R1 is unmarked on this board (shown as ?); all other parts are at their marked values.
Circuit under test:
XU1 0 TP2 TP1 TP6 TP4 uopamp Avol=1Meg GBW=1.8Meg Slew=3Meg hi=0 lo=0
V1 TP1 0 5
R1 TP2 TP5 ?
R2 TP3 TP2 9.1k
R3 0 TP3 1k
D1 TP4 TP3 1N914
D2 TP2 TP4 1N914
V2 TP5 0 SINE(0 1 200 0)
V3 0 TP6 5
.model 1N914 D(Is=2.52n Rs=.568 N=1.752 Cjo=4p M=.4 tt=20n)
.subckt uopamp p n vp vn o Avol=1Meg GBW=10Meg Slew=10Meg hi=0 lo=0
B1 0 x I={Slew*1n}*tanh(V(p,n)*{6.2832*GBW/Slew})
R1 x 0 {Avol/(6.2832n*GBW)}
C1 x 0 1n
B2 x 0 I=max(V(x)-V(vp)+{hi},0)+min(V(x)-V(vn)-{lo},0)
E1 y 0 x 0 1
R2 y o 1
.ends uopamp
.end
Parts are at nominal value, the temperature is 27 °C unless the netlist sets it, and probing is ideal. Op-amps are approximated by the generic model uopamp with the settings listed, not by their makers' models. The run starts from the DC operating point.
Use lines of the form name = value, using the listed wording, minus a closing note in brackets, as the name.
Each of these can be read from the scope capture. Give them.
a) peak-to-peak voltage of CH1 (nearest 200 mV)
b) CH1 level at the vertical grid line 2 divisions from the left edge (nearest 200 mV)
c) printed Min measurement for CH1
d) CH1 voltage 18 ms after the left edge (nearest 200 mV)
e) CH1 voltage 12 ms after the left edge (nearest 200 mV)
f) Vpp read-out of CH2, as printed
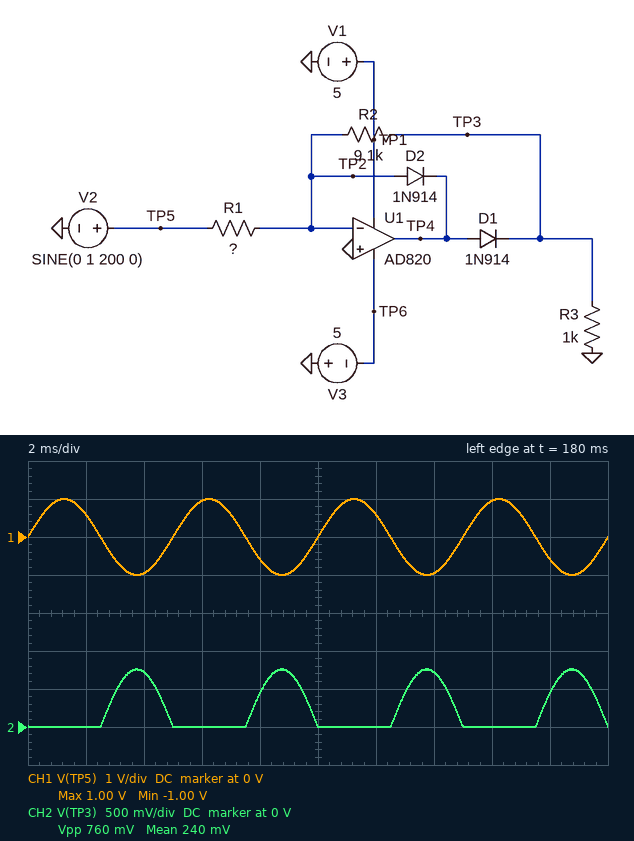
peak-to-peak voltage of CH1 = 2.0 V
CH1 level at the vertical grid line 2 divisions from the left edge = -1.0 V
printed Min measurement for CH1 = -1.00 V
CH1 voltage 18 ms after the left edge = -600 mV
CH1 voltage 12 ms after the left edge = 600 mV
Vpp read-out of CH2, as printed = 760 mV
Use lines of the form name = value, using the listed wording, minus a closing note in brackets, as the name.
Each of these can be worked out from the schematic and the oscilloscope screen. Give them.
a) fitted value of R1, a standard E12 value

fitted value of R1, a standard E12 value = 12 kΩ
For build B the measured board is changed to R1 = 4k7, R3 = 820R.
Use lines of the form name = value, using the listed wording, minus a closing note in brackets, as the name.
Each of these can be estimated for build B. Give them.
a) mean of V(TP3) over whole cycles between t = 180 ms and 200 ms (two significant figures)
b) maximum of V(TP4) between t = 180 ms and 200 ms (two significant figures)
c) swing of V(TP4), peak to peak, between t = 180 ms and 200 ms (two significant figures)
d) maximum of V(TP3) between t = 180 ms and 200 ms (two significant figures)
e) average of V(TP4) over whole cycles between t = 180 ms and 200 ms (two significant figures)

mean of V(TP3) over whole cycles between t = 180 ms and 200 ms = 620 mV
maximum of V(TP4) between t = 180 ms and 200 ms = 2.6 V
swing of V(TP4), peak to peak, between t = 180 ms and 200 ms = 3.1 V
maximum of V(TP3) between t = 180 ms and 200 ms = 1.9 V
average of V(TP4) over whole cycles between t = 180 ms and 200 ms = 670 mV
